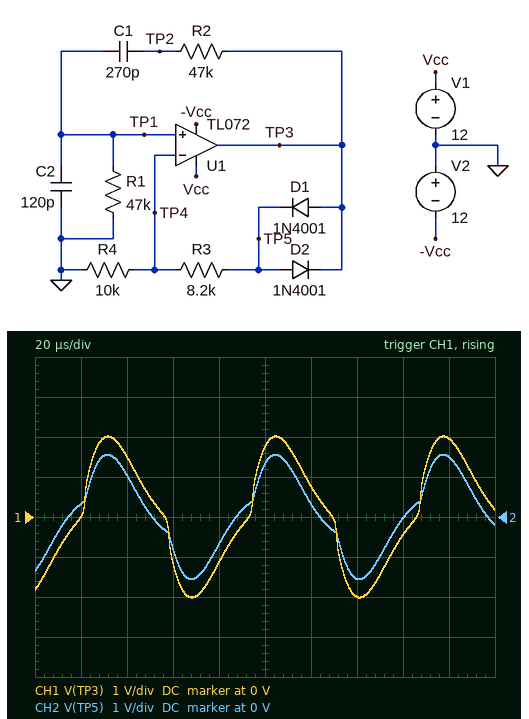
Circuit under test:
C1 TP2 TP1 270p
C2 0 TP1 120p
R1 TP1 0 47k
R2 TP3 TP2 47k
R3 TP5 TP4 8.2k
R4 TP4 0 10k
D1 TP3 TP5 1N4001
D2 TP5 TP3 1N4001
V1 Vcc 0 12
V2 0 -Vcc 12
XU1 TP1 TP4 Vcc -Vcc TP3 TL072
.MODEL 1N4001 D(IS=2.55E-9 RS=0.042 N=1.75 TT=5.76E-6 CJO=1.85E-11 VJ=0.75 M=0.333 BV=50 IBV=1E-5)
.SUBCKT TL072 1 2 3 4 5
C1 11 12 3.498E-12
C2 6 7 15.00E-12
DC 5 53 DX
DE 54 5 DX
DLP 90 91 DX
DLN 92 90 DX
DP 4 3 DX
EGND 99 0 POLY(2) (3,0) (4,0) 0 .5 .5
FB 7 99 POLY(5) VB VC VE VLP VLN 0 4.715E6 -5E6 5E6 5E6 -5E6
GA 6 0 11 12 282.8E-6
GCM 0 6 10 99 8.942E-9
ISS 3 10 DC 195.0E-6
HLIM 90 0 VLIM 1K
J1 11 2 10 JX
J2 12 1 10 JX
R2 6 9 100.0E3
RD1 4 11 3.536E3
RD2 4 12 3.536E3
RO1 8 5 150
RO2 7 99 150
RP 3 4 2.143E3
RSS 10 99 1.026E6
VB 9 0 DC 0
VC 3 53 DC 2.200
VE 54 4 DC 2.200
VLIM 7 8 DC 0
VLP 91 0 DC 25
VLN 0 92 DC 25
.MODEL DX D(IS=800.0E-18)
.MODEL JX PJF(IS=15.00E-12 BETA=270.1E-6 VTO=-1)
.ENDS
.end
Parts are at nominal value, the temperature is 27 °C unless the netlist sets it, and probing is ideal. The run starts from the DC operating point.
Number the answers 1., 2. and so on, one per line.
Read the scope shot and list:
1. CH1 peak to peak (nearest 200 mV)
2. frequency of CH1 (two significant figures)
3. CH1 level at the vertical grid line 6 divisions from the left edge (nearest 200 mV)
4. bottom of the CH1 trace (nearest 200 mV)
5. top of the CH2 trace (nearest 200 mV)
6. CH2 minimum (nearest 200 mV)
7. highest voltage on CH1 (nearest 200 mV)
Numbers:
1. 4.0 V
2. 14 kHz
3. 800 mV
4. -2.0 V
5. 1.6 V
6. -1.6 V
7. 2.0 V
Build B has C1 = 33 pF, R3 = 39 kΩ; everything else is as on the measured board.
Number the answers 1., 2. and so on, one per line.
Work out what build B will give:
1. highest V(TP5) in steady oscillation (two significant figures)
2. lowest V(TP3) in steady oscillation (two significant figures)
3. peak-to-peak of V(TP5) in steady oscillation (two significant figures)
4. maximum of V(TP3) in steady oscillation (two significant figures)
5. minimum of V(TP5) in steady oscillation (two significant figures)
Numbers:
1. 1.5 V
2. -1.9 V
3. 3.0 V
4. 1.9 V
5. -1.5 V
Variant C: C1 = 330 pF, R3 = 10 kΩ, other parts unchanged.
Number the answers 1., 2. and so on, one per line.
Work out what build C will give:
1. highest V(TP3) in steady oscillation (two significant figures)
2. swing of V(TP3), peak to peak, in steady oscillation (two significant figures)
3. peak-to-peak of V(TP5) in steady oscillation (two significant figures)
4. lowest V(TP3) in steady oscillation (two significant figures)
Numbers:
1. 3.5 V
2. 7.1 V
3. 6.1 V
4. -3.5 V
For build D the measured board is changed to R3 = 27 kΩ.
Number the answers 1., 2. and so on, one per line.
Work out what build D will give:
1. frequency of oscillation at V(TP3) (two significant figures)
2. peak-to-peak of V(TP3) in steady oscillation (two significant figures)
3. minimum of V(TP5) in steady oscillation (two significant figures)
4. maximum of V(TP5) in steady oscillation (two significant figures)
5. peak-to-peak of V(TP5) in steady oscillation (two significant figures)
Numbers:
1. 13 kHz
2. 21 V
3. -11 V
4. 11 V
5. 22 V
